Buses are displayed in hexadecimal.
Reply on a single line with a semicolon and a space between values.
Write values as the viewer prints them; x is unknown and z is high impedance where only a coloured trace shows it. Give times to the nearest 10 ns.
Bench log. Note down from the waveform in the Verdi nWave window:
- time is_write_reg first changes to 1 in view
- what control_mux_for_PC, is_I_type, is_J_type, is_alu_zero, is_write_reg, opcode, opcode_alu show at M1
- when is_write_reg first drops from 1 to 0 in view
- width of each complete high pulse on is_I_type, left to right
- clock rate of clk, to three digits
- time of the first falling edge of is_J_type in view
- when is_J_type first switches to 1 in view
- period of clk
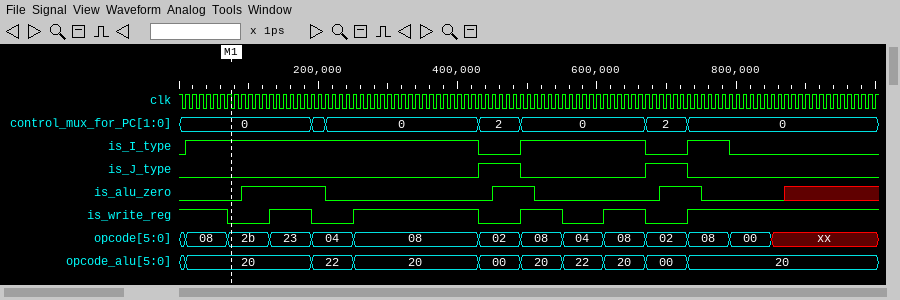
130 ns; control_mux_for_PC=0, is_I_type=1, is_J_type=0, is_alu_zero=0, is_write_reg=0, opcode=2b, opcode_alu=20; 70 ns; 420 ns, 180 ns, 60 ns; 100 MHz; 490 ns; 430 ns; 10 ns
